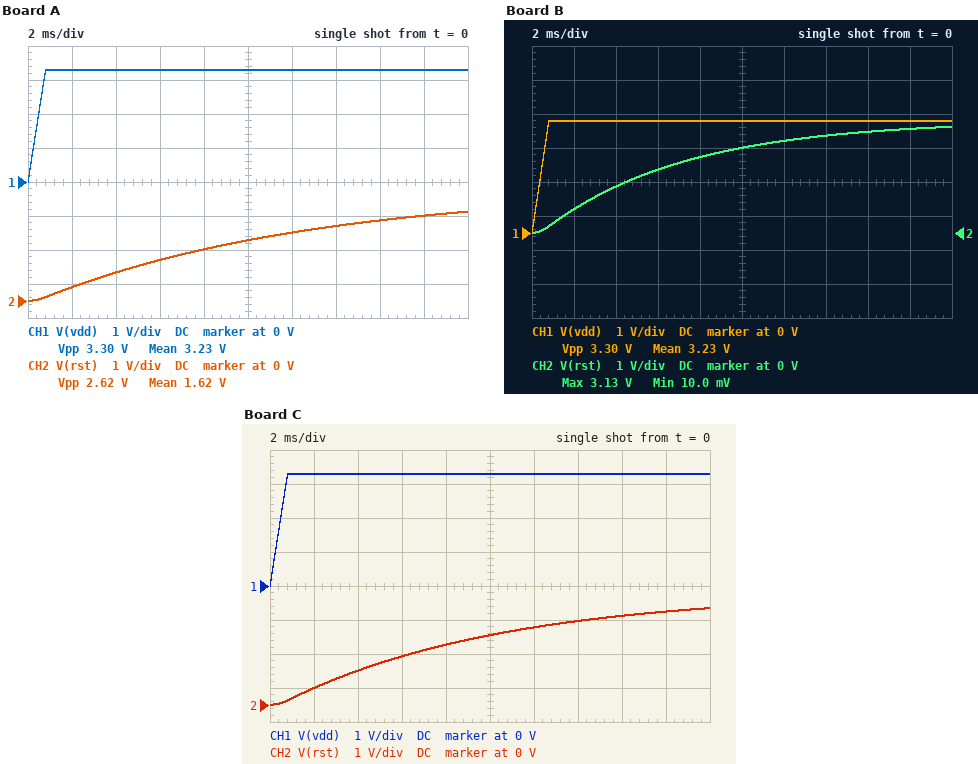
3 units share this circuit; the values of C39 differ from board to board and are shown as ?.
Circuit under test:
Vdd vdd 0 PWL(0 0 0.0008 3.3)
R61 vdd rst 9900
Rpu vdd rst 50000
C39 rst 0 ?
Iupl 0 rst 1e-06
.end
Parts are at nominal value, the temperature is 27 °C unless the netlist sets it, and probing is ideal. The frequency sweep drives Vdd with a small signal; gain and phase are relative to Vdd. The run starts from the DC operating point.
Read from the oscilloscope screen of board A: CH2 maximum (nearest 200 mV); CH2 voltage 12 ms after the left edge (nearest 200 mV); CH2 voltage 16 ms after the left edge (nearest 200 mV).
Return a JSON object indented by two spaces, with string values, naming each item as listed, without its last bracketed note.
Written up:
{
  "CH2 maximum": "2.6 V",
  "CH2 voltage 12 ms after the left edge": "2.0 V",
  "CH2 voltage 16 ms after the left edge": "2.4 V"
}
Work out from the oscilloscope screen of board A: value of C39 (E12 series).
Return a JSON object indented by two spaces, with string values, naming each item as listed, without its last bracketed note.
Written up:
{
  "value of C39": "1.5 µF"
}
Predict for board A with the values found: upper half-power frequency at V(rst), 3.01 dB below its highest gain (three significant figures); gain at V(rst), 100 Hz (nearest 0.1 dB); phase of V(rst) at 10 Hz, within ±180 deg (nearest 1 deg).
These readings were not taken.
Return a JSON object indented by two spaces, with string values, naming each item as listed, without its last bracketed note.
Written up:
{
  "upper half-power frequency at V(rst), 3.01 dB below its highest gain": "12.8 Hz",
  "gain at V(rst), 100 Hz": "-17.9 dB",
  "phase of V(rst) at 10 Hz, within ±180 deg": "-38 deg"
}
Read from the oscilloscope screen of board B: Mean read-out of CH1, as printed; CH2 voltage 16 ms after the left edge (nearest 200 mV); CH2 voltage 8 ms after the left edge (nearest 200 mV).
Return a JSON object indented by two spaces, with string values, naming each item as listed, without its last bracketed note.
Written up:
{
  "Mean read-out of CH1, as printed": "3.23 V",
  "CH2 voltage 16 ms after the left edge": "3.0 V",
  "CH2 voltage 8 ms after the left edge": "2.2 V"
}
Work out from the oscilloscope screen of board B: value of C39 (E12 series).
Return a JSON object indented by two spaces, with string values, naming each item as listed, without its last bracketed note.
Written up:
{
  "value of C39": "820 nF"
}
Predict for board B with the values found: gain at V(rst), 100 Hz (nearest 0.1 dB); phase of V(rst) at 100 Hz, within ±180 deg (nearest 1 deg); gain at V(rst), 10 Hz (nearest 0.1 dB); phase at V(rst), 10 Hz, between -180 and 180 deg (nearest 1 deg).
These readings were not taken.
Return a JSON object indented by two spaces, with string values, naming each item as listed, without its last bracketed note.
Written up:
{
  "gain at V(rst), 100 Hz": "-12.8 dB",
  "phase of V(rst) at 100 Hz, within ±180 deg": "-77 deg",
  "gain at V(rst), 10 Hz": "-0.7 dB",
  "phase at V(rst), 10 Hz, between -180 and 180 deg": "-23 deg"
}
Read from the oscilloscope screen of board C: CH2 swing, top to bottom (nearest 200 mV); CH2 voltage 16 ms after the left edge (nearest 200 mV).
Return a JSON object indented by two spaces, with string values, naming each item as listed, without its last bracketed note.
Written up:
{
  "CH2 swing, top to bottom": "2.8 V",
  "CH2 voltage 16 ms after the left edge": "2.6 V"
}
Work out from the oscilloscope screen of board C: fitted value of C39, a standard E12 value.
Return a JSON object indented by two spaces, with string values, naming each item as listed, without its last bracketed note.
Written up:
{
  "fitted value of C39, a standard E12 value": "1.2 µF"
}
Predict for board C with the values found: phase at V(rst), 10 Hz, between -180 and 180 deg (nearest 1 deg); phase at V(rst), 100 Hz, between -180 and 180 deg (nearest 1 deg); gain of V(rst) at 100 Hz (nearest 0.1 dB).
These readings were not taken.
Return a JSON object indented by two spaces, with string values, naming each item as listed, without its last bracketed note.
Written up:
{
  "phase at V(rst), 10 Hz, between -180 and 180 deg": "-32 deg",
  "phase at V(rst), 100 Hz, between -180 and 180 deg": "-81 deg",
  "gain of V(rst) at 100 Hz": "-16.0 dB"
}
